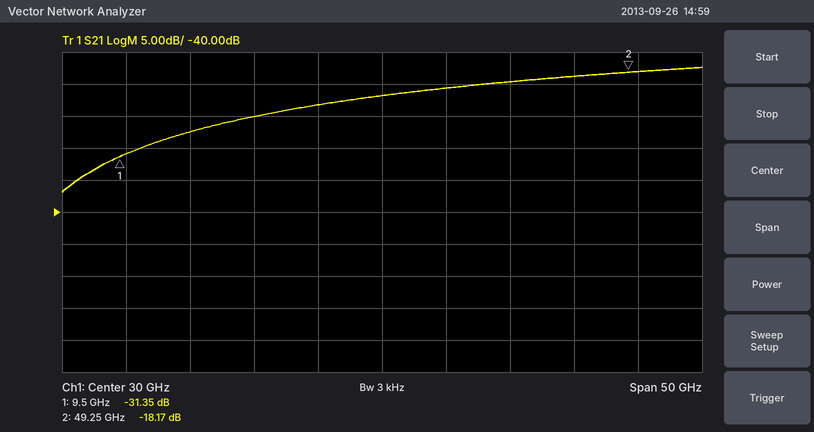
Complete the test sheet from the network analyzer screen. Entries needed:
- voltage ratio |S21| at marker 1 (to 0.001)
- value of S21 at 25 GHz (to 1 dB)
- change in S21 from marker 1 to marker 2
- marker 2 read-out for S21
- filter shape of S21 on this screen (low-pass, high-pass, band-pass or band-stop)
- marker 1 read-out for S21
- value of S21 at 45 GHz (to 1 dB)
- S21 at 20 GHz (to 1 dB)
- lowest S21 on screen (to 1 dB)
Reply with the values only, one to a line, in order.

0.027
-23 dB
13.18 dB
-18.17 dB
high-pass
-31.35 dB
-19 dB
-25 dB
-37 dB
